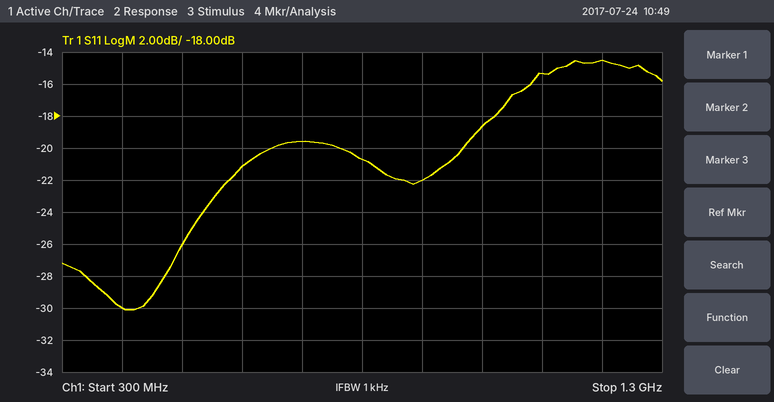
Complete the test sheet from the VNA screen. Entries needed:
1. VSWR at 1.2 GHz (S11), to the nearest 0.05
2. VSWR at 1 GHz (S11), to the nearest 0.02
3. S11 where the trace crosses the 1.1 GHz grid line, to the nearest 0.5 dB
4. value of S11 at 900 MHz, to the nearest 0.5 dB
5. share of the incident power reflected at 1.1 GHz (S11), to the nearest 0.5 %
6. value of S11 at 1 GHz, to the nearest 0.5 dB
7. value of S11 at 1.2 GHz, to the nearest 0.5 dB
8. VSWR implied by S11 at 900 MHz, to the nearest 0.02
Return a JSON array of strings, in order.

["1.45", "1.26", "-15.5 dB", "-22.0 dB", "3.0 %", "-18.5 dB", "-14.5 dB", "1.18"]
